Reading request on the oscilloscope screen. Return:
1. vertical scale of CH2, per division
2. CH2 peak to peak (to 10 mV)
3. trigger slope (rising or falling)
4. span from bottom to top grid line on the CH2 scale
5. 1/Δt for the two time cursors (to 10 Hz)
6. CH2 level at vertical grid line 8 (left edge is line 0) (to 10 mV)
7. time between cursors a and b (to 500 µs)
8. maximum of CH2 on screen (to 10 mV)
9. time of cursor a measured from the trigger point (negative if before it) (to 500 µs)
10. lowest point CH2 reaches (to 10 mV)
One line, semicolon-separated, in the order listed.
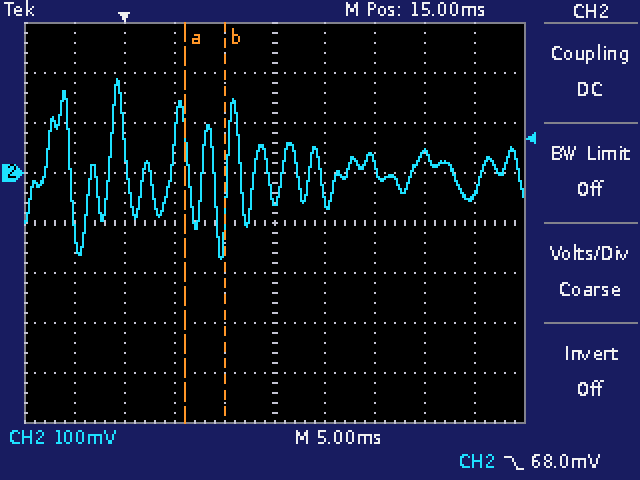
100 mV; 360 mV; falling; 800 mV; 250 Hz; 40 mV; 4.0 ms; 190 mV; +6.0 ms; -170 mV
